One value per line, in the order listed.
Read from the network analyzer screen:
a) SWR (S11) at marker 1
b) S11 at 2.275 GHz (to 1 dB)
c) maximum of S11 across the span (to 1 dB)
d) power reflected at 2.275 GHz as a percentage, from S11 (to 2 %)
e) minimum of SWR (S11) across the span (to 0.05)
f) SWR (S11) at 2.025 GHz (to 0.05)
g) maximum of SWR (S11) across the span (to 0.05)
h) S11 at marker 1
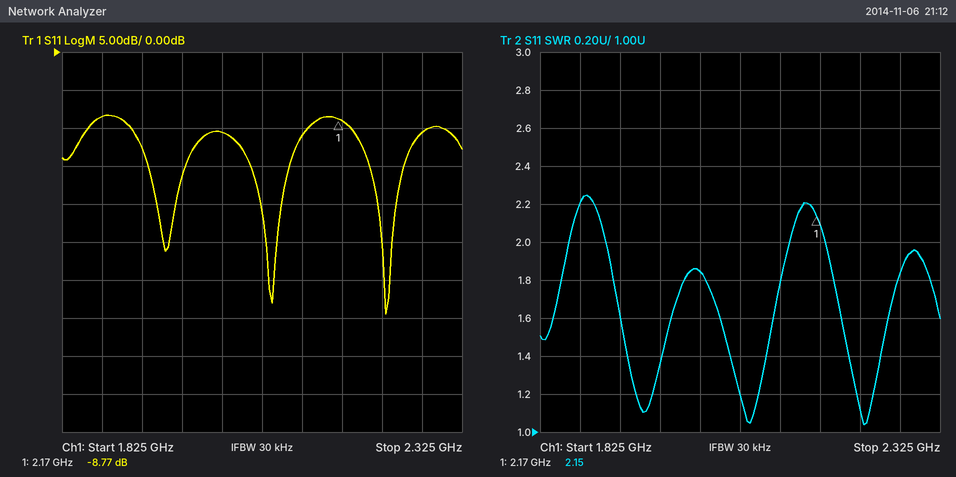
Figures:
2.15
-11 dB
-8 dB
8 %
1.05
1.85
2.25
-8.77 dB
